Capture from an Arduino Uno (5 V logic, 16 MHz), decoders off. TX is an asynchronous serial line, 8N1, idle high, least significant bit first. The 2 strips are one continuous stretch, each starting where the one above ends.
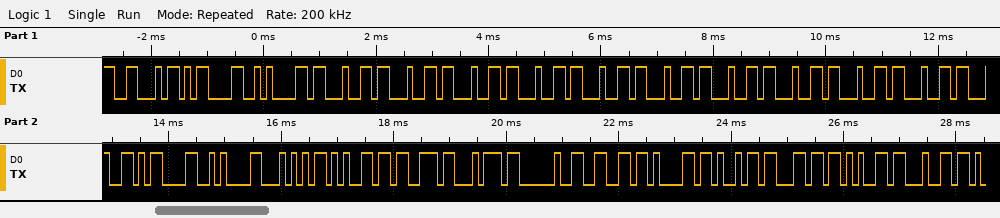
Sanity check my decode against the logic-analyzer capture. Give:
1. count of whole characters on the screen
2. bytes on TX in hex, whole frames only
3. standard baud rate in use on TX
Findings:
27
0x46 0x0D 0x0A 0x23 0x23 0x23 0x23 0x23 0x23 0x23 0x23 0x23 0x23 0x23 0x0D 0x0A 0x54 0x65 0x73 0x74 0x20 0x66 0x61 0x69 0x6C 0x65 0x64
9600 baud
